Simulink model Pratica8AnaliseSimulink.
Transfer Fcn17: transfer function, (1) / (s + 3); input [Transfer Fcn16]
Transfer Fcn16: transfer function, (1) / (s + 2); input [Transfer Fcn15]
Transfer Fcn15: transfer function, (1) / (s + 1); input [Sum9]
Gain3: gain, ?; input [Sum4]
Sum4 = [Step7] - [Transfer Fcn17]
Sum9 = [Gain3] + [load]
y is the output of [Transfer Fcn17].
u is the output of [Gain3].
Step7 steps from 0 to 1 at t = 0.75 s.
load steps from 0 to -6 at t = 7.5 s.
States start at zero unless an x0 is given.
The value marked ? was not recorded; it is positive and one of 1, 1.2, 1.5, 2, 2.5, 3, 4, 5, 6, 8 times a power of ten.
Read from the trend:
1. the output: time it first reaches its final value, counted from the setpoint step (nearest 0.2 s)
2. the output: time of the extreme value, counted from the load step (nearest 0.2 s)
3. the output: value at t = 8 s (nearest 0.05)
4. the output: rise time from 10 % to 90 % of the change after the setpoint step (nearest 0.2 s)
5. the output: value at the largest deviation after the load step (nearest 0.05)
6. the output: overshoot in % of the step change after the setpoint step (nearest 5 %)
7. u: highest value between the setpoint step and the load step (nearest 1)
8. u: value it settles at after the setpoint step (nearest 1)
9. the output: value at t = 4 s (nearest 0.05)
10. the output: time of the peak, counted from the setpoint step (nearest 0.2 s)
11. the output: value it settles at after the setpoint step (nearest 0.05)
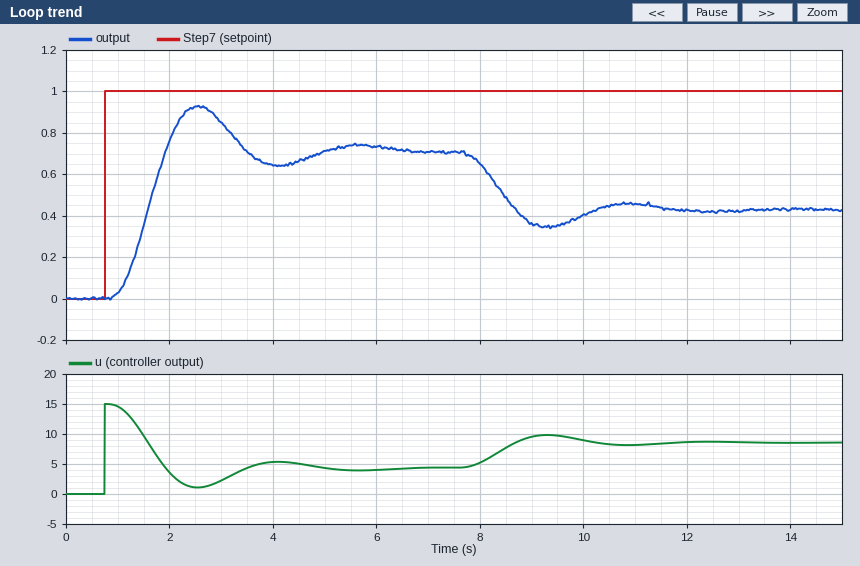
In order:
1.2 s
1.8 s
0.65
0.8 s
0.35
30 %
15
4
0.65
1.8 s
0.70
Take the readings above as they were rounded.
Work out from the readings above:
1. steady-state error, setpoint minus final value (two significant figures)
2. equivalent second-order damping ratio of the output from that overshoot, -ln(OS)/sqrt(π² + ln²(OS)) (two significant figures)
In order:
0.30
0.36
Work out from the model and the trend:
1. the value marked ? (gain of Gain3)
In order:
15
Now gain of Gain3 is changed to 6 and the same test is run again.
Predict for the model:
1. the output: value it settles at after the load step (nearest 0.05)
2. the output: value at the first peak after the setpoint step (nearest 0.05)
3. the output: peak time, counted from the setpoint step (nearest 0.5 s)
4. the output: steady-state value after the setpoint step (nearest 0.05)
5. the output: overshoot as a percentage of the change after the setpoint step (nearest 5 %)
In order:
0.00
0.55
2.5 s
0.50
10 %
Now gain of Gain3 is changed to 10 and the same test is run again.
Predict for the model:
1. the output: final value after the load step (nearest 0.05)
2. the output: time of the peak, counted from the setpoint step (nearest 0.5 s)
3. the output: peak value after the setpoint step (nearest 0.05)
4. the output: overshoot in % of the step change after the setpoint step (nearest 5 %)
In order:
0.25
2.0 s
0.75
20 %
